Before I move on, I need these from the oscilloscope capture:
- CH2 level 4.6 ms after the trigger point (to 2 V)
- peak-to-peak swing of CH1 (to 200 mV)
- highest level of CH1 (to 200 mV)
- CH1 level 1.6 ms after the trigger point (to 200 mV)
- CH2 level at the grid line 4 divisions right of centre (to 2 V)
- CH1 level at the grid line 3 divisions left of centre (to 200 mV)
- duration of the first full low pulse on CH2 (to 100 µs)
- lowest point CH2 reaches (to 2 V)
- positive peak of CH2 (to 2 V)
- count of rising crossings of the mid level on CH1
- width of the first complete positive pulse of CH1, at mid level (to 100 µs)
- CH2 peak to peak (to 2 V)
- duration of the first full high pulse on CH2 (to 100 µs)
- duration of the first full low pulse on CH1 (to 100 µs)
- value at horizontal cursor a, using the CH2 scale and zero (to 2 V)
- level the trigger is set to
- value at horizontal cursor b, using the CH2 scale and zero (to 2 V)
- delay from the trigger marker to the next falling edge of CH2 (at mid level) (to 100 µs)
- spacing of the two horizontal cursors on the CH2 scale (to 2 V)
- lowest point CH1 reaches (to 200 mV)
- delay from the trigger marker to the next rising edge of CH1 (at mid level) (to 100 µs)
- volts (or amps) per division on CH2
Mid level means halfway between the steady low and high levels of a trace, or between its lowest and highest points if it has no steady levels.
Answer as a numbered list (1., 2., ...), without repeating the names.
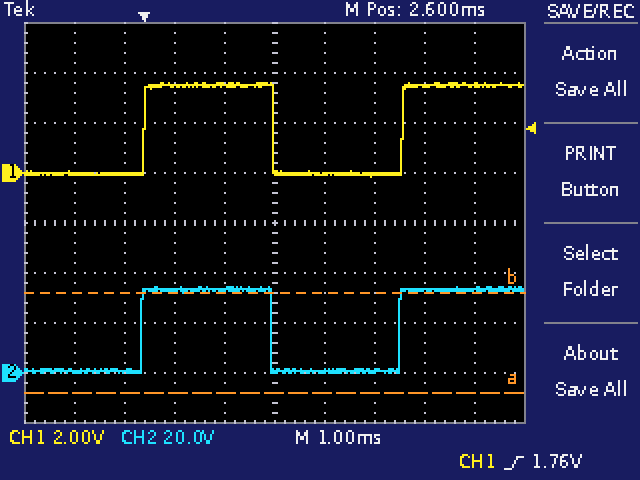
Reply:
1. 0 V
2. 3.8 V
3. 3.6 V
4. 3.6 V
5. 34 V
6. 0.0 V
7. 2.6 ms
8. 0 V
9. 34 V
10. 2
11. 2.6 ms
12. 34 V
13. 2.6 ms
14. 2.6 ms
15. -8 V
16. 1.76 V
17. 32 V
18. 2.5 ms
19. 40 V
20. -200 mV
21. 5.2 ms
22. 20 V
